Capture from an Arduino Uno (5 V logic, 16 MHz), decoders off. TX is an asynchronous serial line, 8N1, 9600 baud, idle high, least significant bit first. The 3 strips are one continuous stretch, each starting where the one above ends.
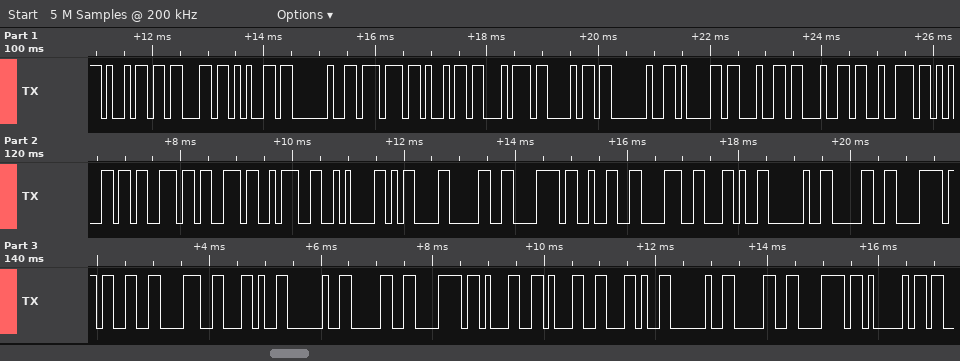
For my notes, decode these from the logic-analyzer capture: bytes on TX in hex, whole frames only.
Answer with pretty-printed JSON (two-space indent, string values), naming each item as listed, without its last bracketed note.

{
  "bytes on TX in hex, whole frames only": "0x69 0x63 0x65 0x20 0x77 0x69 0x74 0x68 0x20 0x61 0x64 0x64 0x72 0x65 0x73 0x73 0x3A 0x0A 0x0D 0x30 0x78 0x32 0x38 0x2C 0x20 0x30 0x78 0x33 0x38 0x2C 0x20 0x30 0x78 0x31 0x31 0x2C 0x20 0x30 0x78 0x41"
}
